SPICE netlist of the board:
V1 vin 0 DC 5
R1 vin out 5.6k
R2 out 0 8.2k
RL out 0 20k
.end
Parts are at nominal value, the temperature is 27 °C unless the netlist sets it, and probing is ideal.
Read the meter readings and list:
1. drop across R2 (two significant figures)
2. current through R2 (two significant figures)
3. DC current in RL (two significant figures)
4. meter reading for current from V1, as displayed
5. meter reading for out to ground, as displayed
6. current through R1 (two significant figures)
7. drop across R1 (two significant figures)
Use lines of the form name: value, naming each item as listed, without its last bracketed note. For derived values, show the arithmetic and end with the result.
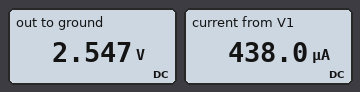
drop across R2: 2.547 V = 2.5 V
current through R2: (2.547 V) / 8.2 kΩ = 310 µA
DC current in RL: (2.547 V) / 20 kΩ = 130 µA
meter reading for current from V1, as displayed: 438.0 µA
meter reading for out to ground, as displayed: 2.547 V
current through R1: (5 V - 2.547 V) / 5.6 kΩ = 440 µA
drop across R1: 5 V - 2.547 V = 2.5 V
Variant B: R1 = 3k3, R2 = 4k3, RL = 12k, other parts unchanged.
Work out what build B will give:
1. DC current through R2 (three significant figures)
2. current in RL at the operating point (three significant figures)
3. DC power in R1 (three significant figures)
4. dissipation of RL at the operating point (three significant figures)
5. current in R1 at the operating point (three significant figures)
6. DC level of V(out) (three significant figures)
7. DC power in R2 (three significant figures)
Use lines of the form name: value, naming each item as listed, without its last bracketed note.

DC current through R2: 569 µA
current in RL at the operating point: 204 µA
DC power in R1: 1.97 mW
dissipation of RL at the operating point: 499 µW
current in R1 at the operating point: 773 µA
DC level of V(out): 2.45 V
DC power in R2: 1.39 mW
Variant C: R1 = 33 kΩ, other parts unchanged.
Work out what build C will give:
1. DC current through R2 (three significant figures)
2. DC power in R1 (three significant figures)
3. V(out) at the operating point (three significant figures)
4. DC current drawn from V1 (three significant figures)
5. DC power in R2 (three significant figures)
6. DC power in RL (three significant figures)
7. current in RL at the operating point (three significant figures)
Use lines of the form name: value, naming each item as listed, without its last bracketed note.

DC current through R2: 91.4 µA
DC power in R1: 548 µW
V(out) at the operating point: 749 mV
DC current drawn from V1: 129 µA
DC power in R2: 68.4 µW
DC power in RL: 28.1 µW
current in RL at the operating point: 37.5 µA
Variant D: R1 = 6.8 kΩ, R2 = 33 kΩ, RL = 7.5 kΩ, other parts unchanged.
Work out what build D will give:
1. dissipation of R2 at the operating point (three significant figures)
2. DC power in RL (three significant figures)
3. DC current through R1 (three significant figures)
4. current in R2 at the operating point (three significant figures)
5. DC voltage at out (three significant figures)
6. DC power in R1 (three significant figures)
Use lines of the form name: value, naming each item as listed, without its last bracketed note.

dissipation of R2 at the operating point: 170 µW
DC power in RL: 747 µW
DC current through R1: 387 µA
current in R2 at the operating point: 71.7 µA
DC voltage at out: 2.37 V
DC power in R1: 1.02 mW
